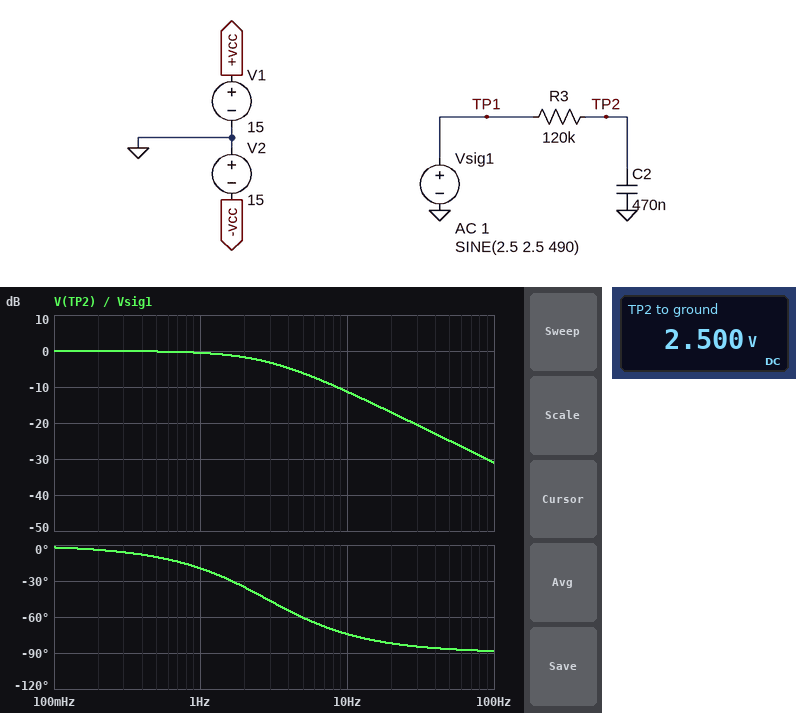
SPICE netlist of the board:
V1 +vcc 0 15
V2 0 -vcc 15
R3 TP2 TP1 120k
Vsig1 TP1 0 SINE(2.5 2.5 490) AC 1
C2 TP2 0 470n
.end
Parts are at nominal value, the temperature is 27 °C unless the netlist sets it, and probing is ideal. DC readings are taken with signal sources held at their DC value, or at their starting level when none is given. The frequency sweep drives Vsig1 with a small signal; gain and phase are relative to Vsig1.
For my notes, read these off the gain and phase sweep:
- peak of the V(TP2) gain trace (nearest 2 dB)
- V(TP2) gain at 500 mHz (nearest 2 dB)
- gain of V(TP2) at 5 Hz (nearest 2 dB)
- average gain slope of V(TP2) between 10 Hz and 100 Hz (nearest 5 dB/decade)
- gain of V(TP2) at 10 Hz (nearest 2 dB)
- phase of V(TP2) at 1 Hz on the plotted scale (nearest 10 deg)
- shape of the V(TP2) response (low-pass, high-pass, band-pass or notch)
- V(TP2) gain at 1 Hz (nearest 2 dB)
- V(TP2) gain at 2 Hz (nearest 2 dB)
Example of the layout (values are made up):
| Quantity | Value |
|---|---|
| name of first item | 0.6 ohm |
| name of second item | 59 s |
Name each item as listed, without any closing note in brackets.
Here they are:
| Quantity | Value |
|---|---|
| peak of the V(TP2) gain trace | 0 dB |
| V(TP2) gain at 500 mHz | 0 dB |
| gain of V(TP2) at 5 Hz | -6 dB |
| average gain slope of V(TP2) between 10 Hz and 100 Hz | -20 dB/decade |
| gain of V(TP2) at 10 Hz | -12 dB |
| phase of V(TP2) at 1 Hz on the plotted scale | -20 deg |
| shape of the V(TP2) response | low-pass |
| V(TP2) gain at 1 Hz | 0 dB |
| V(TP2) gain at 2 Hz | -2 dB |
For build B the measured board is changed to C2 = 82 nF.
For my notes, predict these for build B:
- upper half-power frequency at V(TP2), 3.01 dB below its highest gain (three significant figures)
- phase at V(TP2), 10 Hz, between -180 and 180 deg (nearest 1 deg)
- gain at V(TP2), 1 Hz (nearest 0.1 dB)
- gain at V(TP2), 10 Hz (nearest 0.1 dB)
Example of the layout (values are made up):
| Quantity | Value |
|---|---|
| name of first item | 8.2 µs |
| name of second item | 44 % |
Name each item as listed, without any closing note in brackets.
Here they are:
| Quantity | Value |
|---|---|
| upper half-power frequency at V(TP2), 3.01 dB below its highest gain | 16.2 Hz |
| phase at V(TP2), 10 Hz, between -180 and 180 deg | -32 deg |
| gain at V(TP2), 1 Hz | 0 dB |
| gain at V(TP2), 10 Hz | -1.4 dB |
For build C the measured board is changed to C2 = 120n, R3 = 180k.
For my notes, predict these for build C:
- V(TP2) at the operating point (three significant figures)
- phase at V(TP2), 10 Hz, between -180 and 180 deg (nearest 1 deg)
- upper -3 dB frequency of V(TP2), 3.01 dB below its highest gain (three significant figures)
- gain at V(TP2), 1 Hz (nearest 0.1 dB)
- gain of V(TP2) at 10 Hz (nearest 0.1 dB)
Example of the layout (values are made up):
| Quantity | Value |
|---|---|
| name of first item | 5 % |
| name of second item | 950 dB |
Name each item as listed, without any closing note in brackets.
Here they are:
| Quantity | Value |
|---|---|
| V(TP2) at the operating point | 2.50 V |
| phase at V(TP2), 10 Hz, between -180 and 180 deg | -54 deg |
| upper -3 dB frequency of V(TP2), 3.01 dB below its highest gain | 7.37 Hz |
| gain at V(TP2), 1 Hz | -0.1 dB |
| gain of V(TP2) at 10 Hz | -4.5 dB |
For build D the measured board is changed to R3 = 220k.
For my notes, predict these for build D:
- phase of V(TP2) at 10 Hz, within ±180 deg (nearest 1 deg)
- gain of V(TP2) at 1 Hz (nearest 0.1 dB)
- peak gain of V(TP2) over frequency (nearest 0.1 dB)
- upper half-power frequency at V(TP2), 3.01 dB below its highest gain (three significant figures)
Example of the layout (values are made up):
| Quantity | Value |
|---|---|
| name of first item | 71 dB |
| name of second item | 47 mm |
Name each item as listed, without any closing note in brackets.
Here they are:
| Quantity | Value |
|---|---|
| phase of V(TP2) at 10 Hz, within ±180 deg | -81 deg |
| gain of V(TP2) at 1 Hz | -1.5 dB |
| peak gain of V(TP2) over frequency | 0 dB |
| upper half-power frequency at V(TP2), 3.01 dB below its highest gain | 1.54 Hz |
